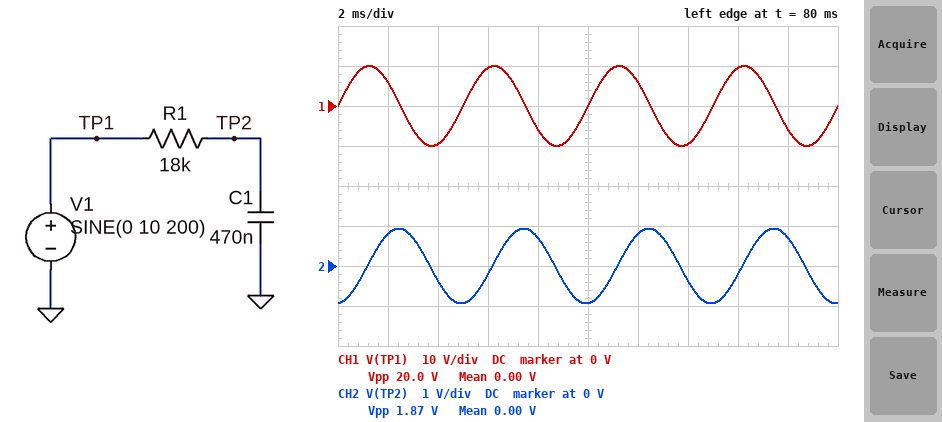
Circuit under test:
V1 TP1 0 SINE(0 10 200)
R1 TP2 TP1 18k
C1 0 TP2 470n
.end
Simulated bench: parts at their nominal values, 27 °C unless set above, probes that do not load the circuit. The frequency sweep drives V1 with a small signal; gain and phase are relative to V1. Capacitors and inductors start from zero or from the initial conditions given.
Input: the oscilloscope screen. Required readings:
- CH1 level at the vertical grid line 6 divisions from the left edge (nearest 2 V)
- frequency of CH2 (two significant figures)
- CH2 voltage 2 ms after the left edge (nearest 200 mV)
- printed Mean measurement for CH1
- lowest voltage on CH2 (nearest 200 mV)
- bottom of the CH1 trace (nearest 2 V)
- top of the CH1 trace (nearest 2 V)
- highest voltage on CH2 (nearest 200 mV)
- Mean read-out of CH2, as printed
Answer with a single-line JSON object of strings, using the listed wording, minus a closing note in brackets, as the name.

{"CH1 level at the vertical grid line 6 divisions from the left edge": "6 V", "frequency of CH2": "200 Hz", "CH2 voltage 2 ms after the left edge": "800 mV", "printed Mean measurement for CH1": "0.00 V", "lowest voltage on CH2": "-1.0 V", "bottom of the CH1 trace": "-10 V", "top of the CH1 trace": "10 V", "highest voltage on CH2": "1.0 V", "Mean read-out of CH2, as printed": "0.00 V"}
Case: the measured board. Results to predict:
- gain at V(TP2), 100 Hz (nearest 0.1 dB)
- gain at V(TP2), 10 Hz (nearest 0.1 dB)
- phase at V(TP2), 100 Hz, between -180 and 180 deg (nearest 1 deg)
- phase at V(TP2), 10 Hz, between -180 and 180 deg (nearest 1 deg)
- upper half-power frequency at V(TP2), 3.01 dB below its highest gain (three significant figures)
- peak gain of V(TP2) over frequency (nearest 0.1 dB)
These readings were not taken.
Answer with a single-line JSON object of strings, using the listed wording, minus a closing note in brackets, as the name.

{"gain at V(TP2), 100 Hz": "-14.7 dB", "gain at V(TP2), 10 Hz": "-1.1 dB", "phase at V(TP2), 100 Hz, between -180 and 180 deg": "-79 deg", "phase at V(TP2), 10 Hz, between -180 and 180 deg": "-28 deg", "upper half-power frequency at V(TP2), 3.01 dB below its highest gain": "18.8 Hz", "peak gain of V(TP2) over frequency": "0 dB"}
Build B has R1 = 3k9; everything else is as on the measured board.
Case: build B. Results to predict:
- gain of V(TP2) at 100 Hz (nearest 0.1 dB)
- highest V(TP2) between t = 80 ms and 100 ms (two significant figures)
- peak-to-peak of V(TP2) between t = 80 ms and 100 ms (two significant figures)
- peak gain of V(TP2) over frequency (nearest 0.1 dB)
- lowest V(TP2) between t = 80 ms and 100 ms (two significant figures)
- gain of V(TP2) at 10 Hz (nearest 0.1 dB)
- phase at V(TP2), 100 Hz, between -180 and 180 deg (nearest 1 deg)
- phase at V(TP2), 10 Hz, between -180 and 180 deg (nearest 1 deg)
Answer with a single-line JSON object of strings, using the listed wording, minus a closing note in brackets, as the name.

{"gain of V(TP2) at 100 Hz": "-3.7 dB", "highest V(TP2) between t = 80 ms and 100 ms": "4.0 V", "peak-to-peak of V(TP2) between t = 80 ms and 100 ms": "8.0 V", "peak gain of V(TP2) over frequency": "0 dB", "lowest V(TP2) between t = 80 ms and 100 ms": "-4.0 V", "gain of V(TP2) at 10 Hz": "-0.1 dB", "phase at V(TP2), 100 Hz, between -180 and 180 deg": "-49 deg", "phase at V(TP2), 10 Hz, between -180 and 180 deg": "-7 deg"}
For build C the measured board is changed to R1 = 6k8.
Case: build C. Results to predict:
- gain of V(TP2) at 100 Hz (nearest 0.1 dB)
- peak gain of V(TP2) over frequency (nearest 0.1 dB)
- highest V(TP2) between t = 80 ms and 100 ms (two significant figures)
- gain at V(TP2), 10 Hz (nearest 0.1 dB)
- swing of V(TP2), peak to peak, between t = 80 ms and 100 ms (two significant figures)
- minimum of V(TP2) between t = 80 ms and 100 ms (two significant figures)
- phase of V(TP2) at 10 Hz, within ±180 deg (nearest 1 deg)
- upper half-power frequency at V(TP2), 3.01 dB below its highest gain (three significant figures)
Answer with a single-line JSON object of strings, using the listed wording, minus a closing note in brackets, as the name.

{"gain of V(TP2) at 100 Hz": "-7.0 dB", "peak gain of V(TP2) over frequency": "0 dB", "highest V(TP2) between t = 80 ms and 100 ms": "2.4 V", "gain at V(TP2), 10 Hz": "-0.2 dB", "swing of V(TP2), peak to peak, between t = 80 ms and 100 ms": "4.8 V", "minimum of V(TP2) between t = 80 ms and 100 ms": "-2.4 V", "phase of V(TP2) at 10 Hz, within ±180 deg": "-11 deg", "upper half-power frequency at V(TP2), 3.01 dB below its highest gain": "49.8 Hz"}
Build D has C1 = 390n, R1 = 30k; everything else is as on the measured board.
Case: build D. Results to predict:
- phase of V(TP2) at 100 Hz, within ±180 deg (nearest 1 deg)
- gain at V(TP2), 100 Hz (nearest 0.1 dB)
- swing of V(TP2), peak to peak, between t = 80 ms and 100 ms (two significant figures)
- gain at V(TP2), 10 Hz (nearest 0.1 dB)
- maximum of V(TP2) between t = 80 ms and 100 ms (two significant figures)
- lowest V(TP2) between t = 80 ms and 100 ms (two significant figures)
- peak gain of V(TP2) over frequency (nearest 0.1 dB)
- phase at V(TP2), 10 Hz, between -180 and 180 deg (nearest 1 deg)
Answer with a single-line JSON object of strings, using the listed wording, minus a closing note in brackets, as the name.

{"phase of V(TP2) at 100 Hz, within ±180 deg": "-82 deg", "gain at V(TP2), 100 Hz": "-17.4 dB", "swing of V(TP2), peak to peak, between t = 80 ms and 100 ms": "1.4 V", "gain at V(TP2), 10 Hz": "-1.9 dB", "maximum of V(TP2) between t = 80 ms and 100 ms": "680 mV", "lowest V(TP2) between t = 80 ms and 100 ms": "-680 mV", "peak gain of V(TP2) over frequency": "0 dB", "phase at V(TP2), 10 Hz, between -180 and 180 deg": "-36 deg"}
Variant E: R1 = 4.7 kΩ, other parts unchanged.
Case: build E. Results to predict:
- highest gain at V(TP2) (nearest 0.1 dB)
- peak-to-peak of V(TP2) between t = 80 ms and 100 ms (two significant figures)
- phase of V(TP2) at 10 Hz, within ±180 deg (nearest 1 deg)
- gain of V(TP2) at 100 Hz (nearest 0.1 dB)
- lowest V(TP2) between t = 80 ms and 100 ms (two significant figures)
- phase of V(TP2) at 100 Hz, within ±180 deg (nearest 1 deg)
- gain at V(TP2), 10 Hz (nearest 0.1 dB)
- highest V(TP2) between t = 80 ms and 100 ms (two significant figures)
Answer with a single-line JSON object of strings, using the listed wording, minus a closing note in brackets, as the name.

{"highest gain at V(TP2)": "0 dB", "peak-to-peak of V(TP2) between t = 80 ms and 100 ms": "6.8 V", "phase of V(TP2) at 10 Hz, within ±180 deg": "-8 deg", "gain of V(TP2) at 100 Hz": "-4.7 dB", "lowest V(TP2) between t = 80 ms and 100 ms": "-3.4 V", "phase of V(TP2) at 100 Hz, within ±180 deg": "-54 deg", "gain at V(TP2), 10 Hz": "-0.1 dB", "highest V(TP2) between t = 80 ms and 100 ms": "3.4 V"}
